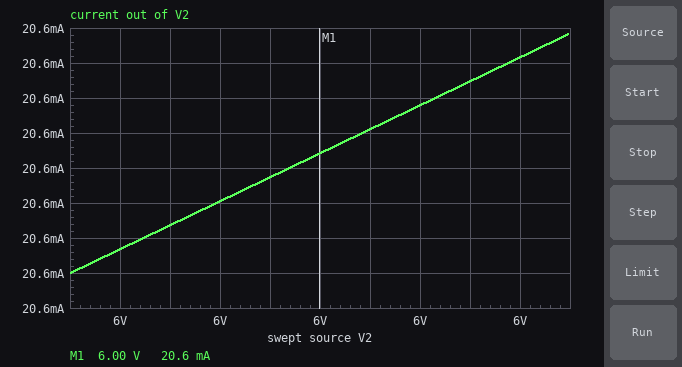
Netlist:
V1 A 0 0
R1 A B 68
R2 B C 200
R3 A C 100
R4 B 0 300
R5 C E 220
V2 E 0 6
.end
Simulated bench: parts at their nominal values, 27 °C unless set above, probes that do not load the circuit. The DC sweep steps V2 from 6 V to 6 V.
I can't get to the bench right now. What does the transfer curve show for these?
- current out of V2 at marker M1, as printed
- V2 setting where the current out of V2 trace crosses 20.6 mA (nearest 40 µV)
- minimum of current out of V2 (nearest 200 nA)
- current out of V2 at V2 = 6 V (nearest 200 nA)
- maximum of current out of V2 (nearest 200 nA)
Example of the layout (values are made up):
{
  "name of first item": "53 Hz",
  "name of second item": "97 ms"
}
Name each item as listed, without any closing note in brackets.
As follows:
{
  "current out of V2 at marker M1, as printed": "20.6 mA",
  "V2 setting where the current out of V2 trace crosses 20.6 mA": "5.99988 V",
  "minimum of current out of V2": "20.5540 mA",
  "current out of V2 at V2 = 6 V": "20.5588 mA",
  "maximum of current out of V2": "20.5608 mA"
}
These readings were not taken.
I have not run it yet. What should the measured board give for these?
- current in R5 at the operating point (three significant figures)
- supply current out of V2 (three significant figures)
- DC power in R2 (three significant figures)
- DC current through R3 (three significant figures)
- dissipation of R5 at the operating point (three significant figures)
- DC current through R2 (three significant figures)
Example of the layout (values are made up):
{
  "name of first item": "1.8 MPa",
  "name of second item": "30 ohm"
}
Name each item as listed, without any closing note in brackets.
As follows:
{
  "current in R5 at the operating point": "20.6 mA",
  "supply current out of V2": "20.6 mA",
  "DC power in R2": "6.69 mW",
  "DC current through R3": "14.8 mA",
  "dissipation of R5 at the operating point": "93.0 mW",
  "DC current through R2": "5.78 mA"
}
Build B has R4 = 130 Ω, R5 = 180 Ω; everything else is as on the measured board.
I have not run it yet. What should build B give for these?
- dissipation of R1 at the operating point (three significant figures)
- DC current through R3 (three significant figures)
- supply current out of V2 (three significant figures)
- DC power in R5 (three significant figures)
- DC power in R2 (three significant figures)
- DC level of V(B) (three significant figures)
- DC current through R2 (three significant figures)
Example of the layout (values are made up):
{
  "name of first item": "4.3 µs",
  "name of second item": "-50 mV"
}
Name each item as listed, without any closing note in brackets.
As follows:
{
  "dissipation of R1 at the operating point": "1.41 mW",
  "DC current through R3": "17.0 mA",
  "supply current out of V2": "23.9 mA",
  "DC power in R5": "103 mW",
  "DC power in R2": "9.62 mW",
  "DC level of V(B)": "310 mV",
  "DC current through R2": "6.94 mA"
}
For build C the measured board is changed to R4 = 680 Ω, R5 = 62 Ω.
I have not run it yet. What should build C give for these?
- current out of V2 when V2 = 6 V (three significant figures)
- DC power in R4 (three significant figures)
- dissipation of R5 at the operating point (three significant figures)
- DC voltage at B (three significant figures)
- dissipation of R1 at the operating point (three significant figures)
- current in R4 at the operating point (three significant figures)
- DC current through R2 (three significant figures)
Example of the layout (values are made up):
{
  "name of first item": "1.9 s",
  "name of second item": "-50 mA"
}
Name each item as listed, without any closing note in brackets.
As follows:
{
  "current out of V2 when V2 = 6 V": "44.7 mA",
  "DC power in R4": "856 µW",
  "dissipation of R5 at the operating point": "124 mW",
  "DC voltage at B": "763 mV",
  "dissipation of R1 at the operating point": "8.56 mW",
  "current in R4 at the operating point": "1.12 mA",
  "DC current through R2": "12.3 mA"
}
